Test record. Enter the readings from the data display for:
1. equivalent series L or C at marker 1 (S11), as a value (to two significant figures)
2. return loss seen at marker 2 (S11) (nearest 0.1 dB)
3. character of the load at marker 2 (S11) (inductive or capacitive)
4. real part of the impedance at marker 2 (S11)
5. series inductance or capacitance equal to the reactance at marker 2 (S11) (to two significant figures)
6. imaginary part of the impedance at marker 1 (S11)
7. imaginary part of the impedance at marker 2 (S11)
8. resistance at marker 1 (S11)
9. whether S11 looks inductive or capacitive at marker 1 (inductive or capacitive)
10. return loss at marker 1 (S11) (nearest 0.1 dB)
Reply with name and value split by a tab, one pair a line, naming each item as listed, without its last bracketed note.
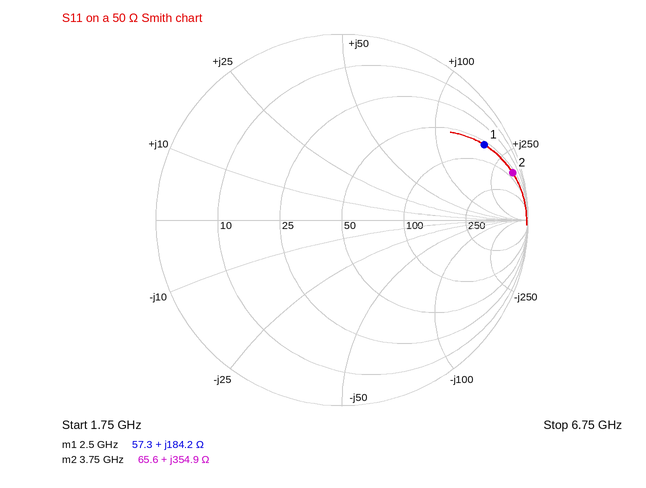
equivalent series L or C at marker 1 (S11), as a value	12 nH
return loss seen at marker 2 (S11)	0.4 dB
character of the load at marker 2 (S11)	inductive
real part of the impedance at marker 2	65.6 Ω
series inductance or capacitance equal to the reactance at marker 2 (S11)	15 nH
imaginary part of the impedance at marker 1	+184.2 Ω
imaginary part of the impedance at marker 2	+354.9 Ω
resistance at marker 1	57.3 Ω
whether S11 looks inductive or capacitive at marker 1	inductive
return loss at marker 1 (S11)	1.3 dB
